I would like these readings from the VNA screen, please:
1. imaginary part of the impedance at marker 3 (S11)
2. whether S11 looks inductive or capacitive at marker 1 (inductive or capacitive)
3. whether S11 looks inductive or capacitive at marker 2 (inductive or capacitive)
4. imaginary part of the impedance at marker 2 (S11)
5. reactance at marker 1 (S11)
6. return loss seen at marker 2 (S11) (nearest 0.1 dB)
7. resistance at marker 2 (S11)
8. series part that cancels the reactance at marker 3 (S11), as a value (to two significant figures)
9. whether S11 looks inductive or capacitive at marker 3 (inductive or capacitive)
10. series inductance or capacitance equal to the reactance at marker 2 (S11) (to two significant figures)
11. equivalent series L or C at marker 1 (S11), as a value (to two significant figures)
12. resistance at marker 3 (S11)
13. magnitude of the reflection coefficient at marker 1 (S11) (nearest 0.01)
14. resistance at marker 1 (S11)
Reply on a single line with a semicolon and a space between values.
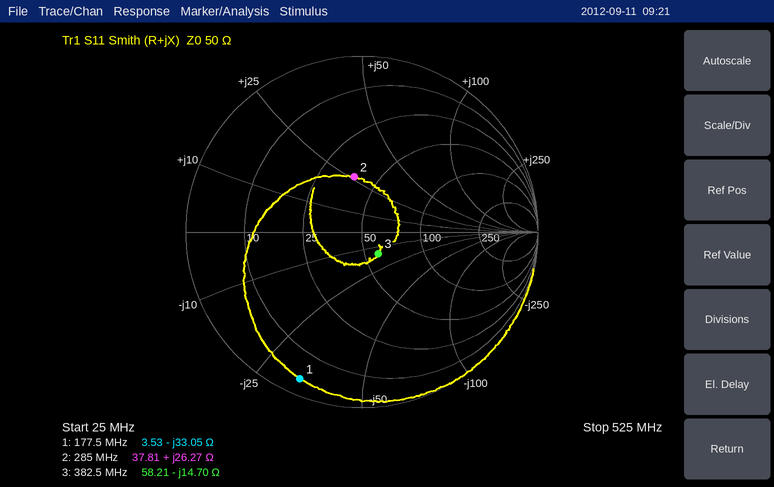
-14.70 Ω; capacitive; inductive; +26.27 Ω; -33.05 Ω; 10.0 dB; 37.81 Ω; 6.1 nH; capacitive; 15 nH; 27 pF; 58.21 Ω; 0.91; 3.53 Ω
